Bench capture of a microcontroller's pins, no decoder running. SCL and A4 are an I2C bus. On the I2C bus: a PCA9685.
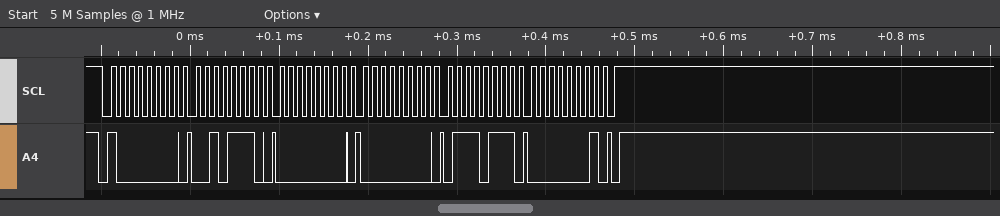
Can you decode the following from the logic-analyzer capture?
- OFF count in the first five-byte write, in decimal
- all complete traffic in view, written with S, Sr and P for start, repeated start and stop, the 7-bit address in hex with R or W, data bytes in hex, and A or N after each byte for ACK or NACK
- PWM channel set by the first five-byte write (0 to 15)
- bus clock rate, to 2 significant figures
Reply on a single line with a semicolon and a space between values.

375; S 40W A 2E A 00 A 00 A 77 A 01 A P; 10; 100 kHz
